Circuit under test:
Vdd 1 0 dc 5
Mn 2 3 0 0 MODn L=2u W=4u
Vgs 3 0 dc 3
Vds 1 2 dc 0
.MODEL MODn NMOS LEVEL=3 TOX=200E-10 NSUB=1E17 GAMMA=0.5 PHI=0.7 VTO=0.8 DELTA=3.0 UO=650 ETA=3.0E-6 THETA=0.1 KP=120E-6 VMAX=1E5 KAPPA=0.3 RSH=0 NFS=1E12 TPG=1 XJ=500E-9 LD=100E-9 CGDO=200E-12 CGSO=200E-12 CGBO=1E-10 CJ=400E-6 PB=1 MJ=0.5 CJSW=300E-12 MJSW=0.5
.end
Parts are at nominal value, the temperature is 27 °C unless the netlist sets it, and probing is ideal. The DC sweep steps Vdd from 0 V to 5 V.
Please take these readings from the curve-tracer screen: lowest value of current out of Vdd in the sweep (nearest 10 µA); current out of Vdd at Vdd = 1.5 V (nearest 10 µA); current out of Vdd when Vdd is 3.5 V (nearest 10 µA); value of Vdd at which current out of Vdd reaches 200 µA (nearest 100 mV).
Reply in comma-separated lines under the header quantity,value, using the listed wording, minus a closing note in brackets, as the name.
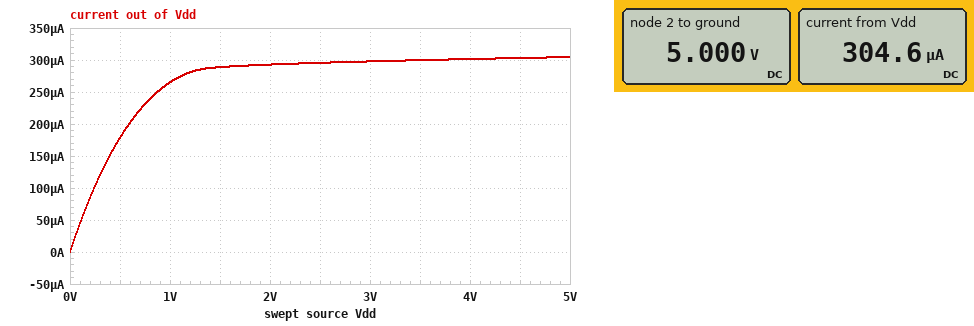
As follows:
quantity,value
lowest value of current out of Vdd in the sweep,0 A
current out of Vdd at Vdd = 1.5 V,290 µA
current out of Vdd when Vdd is 3.5 V,300 µA
value of Vdd at which current out of Vdd reaches 200 µA,600 mV
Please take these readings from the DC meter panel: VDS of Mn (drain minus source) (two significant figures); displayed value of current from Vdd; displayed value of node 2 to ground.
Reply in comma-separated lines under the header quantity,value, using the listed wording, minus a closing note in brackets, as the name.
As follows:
quantity,value
VDS of Mn (drain minus source),5.0 V
displayed value of current from Vdd,304.6 µA
displayed value of node 2 to ground,5.000 V
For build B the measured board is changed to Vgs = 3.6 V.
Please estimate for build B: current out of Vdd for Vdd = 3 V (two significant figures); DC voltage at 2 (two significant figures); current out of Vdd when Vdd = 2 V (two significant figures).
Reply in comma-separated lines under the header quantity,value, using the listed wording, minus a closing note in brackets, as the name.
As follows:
quantity,value
current out of Vdd for Vdd = 3 V,430 µA
DC voltage at 2,5.0 V
current out of Vdd when Vdd = 2 V,420 µA
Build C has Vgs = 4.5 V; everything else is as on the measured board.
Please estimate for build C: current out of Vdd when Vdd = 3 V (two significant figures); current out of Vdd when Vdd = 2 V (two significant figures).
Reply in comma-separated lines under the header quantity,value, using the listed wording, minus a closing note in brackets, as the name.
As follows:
quantity,value
current out of Vdd when Vdd = 3 V,650 µA
current out of Vdd when Vdd = 2 V,630 µA
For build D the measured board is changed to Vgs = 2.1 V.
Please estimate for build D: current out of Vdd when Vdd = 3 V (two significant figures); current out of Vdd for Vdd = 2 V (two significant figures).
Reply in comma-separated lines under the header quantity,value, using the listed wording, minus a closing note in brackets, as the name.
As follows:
quantity,value
current out of Vdd when Vdd = 3 V,130 µA
current out of Vdd for Vdd = 2 V,120 µA
